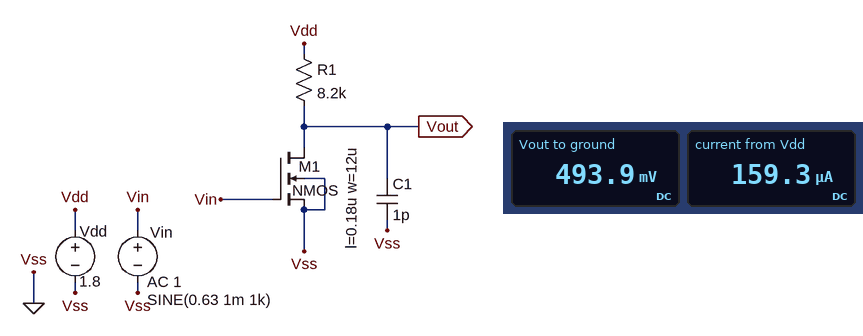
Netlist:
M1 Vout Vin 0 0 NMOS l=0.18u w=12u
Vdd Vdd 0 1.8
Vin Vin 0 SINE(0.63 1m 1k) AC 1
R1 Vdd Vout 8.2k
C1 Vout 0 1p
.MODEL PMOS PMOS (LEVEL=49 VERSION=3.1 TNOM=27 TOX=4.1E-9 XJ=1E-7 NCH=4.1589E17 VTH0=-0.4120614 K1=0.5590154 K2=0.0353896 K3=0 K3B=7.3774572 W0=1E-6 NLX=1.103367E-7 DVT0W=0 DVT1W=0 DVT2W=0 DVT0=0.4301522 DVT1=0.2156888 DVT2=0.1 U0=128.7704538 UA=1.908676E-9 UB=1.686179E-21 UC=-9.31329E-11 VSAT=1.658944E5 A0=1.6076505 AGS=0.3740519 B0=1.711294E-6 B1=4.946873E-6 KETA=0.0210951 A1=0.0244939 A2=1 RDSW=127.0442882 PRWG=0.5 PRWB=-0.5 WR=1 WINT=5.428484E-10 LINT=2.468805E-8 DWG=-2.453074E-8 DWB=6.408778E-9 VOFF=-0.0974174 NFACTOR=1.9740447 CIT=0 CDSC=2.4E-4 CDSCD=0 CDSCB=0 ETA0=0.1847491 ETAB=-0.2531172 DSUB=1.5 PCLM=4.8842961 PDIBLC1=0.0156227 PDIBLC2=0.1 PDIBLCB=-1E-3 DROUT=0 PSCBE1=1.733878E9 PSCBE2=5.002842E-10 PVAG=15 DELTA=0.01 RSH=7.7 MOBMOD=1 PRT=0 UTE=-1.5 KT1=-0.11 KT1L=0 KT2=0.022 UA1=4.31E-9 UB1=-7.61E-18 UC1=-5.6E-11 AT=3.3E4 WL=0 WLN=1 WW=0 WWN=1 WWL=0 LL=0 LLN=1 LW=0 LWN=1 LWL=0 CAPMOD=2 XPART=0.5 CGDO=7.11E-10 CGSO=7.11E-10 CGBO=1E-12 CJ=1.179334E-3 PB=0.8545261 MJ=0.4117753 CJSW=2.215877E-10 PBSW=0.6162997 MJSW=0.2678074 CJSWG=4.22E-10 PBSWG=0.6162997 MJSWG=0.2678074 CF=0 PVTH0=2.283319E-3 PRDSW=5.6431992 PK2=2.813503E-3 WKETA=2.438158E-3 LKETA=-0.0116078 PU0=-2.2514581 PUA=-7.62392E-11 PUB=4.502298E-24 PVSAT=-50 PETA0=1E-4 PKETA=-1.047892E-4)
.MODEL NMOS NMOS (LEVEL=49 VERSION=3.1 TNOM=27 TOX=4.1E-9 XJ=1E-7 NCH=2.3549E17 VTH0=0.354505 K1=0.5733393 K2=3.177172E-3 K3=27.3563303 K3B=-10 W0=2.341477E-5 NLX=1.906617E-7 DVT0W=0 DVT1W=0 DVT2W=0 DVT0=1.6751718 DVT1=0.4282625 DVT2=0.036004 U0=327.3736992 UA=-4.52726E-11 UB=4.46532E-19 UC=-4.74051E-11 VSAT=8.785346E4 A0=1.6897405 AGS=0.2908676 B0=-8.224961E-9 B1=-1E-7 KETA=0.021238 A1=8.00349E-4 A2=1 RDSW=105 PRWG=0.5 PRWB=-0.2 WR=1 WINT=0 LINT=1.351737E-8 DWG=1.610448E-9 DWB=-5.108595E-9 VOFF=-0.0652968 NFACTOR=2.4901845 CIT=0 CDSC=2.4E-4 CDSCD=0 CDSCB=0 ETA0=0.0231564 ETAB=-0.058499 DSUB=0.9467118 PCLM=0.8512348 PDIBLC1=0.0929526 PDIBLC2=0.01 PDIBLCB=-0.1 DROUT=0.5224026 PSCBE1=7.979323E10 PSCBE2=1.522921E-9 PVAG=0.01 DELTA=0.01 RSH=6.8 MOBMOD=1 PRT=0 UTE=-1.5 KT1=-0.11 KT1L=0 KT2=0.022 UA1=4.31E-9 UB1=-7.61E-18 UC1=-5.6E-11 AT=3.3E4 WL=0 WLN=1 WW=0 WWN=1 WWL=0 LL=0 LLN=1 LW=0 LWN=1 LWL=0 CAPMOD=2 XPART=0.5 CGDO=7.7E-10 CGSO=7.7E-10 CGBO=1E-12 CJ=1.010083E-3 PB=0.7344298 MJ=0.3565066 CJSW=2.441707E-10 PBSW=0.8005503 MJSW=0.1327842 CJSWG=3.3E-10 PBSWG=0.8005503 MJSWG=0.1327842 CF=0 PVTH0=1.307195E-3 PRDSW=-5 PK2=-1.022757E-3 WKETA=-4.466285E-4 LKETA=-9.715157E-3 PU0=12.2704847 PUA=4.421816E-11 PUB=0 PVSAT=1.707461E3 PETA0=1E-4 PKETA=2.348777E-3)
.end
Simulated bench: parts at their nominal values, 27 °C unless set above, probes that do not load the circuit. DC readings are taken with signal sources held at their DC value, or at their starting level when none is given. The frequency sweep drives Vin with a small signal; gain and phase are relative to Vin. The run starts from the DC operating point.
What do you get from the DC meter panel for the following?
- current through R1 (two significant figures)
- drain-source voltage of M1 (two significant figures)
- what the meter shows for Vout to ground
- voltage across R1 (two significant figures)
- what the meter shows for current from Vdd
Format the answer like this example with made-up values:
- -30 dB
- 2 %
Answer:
- 160 µA
- 490 mV
- 493.9 mV
- 1.3 V
- 159.3 µA
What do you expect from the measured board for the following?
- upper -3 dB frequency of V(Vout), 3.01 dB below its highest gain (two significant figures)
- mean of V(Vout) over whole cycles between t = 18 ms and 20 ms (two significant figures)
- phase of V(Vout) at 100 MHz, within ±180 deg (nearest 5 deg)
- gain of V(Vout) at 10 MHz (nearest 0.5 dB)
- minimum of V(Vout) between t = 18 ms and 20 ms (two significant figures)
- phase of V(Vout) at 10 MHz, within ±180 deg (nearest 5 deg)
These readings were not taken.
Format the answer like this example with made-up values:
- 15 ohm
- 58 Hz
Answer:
- 28 MHz
- 490 mV
- 105 deg
- 21.5 dB
- 480 mV
- 160 deg
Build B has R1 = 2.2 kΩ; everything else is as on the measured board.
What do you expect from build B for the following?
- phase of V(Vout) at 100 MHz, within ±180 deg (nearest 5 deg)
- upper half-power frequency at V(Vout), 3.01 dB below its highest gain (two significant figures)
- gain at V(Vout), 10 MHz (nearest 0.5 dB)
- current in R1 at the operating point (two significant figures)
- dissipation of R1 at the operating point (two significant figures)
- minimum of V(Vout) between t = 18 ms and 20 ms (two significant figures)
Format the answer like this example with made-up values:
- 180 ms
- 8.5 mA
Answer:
- 130 deg
- 80 MHz
- 14.5 dB
- 210 µA
- 93 µW
- 1.3 V
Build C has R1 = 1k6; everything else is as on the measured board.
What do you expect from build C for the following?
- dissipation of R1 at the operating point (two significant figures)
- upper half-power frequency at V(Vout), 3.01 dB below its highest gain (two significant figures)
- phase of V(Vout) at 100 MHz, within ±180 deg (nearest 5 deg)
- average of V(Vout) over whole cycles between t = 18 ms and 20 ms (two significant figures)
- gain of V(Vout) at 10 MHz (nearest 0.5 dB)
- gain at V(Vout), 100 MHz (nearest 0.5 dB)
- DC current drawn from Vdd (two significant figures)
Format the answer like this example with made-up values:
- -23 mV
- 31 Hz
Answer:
- 72 µW
- 110 MHz
- 135 deg
- 1.5 V
- 12.0 dB
- 9.5 dB
- 210 µA
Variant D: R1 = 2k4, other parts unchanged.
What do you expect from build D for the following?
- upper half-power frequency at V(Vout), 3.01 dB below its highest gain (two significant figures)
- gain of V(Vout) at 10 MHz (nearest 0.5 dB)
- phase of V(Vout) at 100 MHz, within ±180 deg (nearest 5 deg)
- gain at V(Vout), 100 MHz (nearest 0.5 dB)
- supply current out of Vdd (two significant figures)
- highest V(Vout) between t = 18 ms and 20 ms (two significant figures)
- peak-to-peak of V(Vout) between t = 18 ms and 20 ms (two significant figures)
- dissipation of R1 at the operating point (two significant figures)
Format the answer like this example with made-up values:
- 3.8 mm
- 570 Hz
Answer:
- 74 MHz
- 15.0 dB
- 125 deg
- 10.5 dB
- 200 µA
- 1.3 V
- 11 mV
- 100 µW
